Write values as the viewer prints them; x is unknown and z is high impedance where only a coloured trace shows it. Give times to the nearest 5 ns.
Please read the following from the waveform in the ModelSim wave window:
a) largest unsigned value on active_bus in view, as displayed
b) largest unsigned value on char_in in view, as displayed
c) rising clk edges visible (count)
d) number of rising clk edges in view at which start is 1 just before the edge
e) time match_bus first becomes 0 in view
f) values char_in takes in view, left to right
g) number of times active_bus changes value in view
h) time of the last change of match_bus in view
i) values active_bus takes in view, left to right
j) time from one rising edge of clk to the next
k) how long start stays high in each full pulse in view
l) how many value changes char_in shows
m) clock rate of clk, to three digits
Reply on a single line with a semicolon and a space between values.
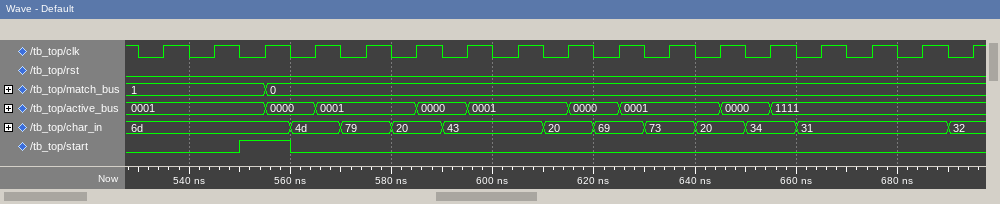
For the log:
1111; 79; 17; 1; 555 ns; 6d, 4d, 79, 20, 43, 20, 69, 73, 20, 34, 31, 32; 8; 555 ns; 0001, 0000, 0001, 0000, 0001, 0000, 0001, 0000, 1111; 10 ns; 10 ns; 11; 100 MHz
